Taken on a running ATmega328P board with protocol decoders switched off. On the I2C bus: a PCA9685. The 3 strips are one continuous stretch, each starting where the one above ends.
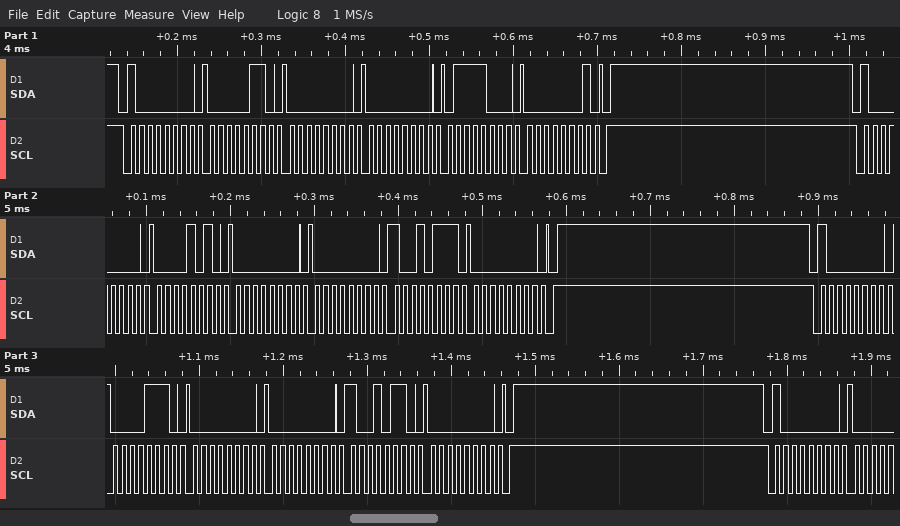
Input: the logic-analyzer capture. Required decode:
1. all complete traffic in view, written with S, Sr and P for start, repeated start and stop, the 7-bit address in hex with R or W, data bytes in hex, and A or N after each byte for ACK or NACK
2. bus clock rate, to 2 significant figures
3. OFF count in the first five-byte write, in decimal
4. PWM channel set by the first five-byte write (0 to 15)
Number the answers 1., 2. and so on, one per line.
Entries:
1. S 40W A 06 A 00 A 00 A 78 A 01 A P S 40W A 0A A 00 A 00 A 97 A 00 A P S 40W A 0E A 00 A 00 A 96 A 00 A P S 40W A
2. 100 kHz
3. 376
4. 0
